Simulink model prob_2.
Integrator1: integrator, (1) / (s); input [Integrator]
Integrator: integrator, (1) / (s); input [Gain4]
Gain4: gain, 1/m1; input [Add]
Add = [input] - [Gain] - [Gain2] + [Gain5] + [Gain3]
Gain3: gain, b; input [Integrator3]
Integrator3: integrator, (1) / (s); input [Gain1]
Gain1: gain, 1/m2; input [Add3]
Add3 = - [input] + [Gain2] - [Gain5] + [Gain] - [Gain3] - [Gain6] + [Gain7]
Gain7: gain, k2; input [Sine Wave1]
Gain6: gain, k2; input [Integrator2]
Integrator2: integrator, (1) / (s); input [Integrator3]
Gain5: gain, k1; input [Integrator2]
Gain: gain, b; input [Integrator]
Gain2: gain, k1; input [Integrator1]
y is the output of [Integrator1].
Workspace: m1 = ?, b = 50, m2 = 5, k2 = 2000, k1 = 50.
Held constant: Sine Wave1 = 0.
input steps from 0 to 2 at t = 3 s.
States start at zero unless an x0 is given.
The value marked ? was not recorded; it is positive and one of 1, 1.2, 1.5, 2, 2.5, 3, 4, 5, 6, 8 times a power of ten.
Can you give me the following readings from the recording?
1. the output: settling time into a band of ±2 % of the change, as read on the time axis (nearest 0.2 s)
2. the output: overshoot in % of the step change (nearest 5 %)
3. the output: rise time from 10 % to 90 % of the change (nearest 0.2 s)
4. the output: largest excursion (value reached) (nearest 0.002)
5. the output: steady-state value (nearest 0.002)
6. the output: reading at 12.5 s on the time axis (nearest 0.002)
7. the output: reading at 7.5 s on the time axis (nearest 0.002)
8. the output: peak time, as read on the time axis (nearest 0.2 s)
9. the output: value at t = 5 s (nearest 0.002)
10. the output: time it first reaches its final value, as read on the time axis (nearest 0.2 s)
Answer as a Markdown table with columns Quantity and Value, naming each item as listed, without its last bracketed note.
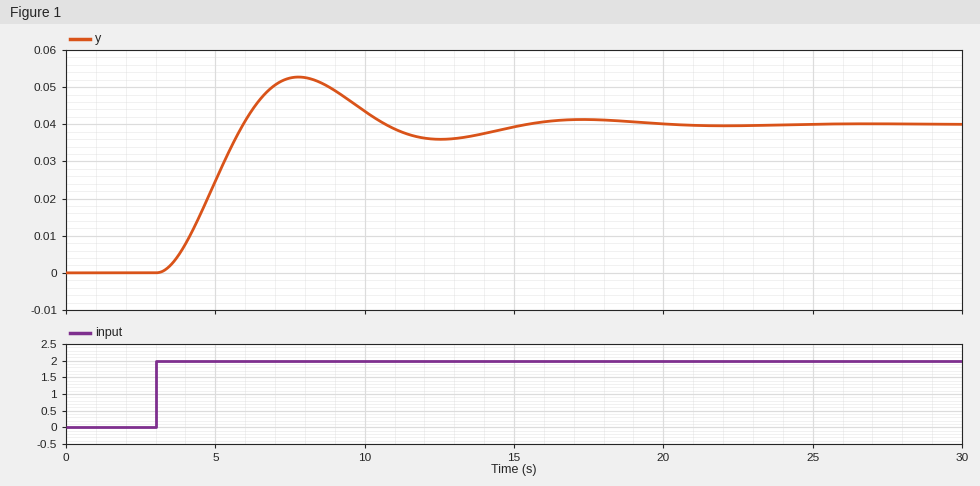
| Quantity | Value |
|---|---|
| the output: settling time into a band of ±2 % of the change, as read on the time axis | 18.8 s |
| the output: overshoot in % of the step change | 30 % |
| the output: rise time from 10 % to 90 % of the change | 2.0 s |
| the output: largest excursion (value reached) | 0.052 |
| the output: steady-state value | 0.040 |
| the output: reading at 12.5 s on the time axis | 0.036 |
| the output: reading at 7.5 s on the time axis | 0.052 |
| the output: peak time, as read on the time axis | 7.8 s |
| the output: value at t = 5 s | 0.024 |
| the output: time it first reaches its final value, as read on the time axis | 6.0 s |
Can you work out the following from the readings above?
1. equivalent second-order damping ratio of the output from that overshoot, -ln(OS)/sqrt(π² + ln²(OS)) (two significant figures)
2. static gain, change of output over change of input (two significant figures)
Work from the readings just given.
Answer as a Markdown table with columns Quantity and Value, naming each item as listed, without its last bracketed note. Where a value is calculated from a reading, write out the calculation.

| Quantity | Value |
|---|---|
| equivalent second-order damping ratio of the output from that overshoot, -ln(OS)/sqrt(π² + ln²(OS)) | ln(0.3) = -1.204; 1.204 / sqrt(9.870 + 1.450) = 0.36 |
| static gain, change of output over change of input | (0.04 - 0) / (2 - 0) = 0.020 |
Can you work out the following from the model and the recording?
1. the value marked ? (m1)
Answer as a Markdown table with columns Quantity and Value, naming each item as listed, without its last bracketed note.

| Quantity | Value |
|---|---|
| the value marked ? | 100 |
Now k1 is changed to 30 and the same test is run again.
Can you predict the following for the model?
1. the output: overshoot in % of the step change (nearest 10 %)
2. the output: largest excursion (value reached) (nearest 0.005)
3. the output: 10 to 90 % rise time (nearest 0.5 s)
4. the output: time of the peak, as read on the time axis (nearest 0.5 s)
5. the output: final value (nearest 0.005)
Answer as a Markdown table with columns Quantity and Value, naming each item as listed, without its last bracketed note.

| Quantity | Value |
|---|---|
| the output: overshoot in % of the step change | 20 % |
| the output: largest excursion (value reached) | 0.080 |
| the output: 10 to 90 % rise time | 3.0 s |
| the output: time of the peak, as read on the time axis | 9.5 s |
| the output: final value | 0.065 |
